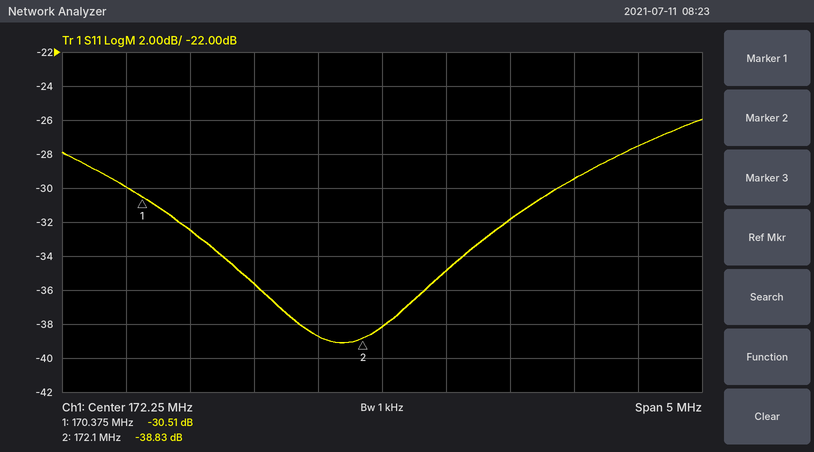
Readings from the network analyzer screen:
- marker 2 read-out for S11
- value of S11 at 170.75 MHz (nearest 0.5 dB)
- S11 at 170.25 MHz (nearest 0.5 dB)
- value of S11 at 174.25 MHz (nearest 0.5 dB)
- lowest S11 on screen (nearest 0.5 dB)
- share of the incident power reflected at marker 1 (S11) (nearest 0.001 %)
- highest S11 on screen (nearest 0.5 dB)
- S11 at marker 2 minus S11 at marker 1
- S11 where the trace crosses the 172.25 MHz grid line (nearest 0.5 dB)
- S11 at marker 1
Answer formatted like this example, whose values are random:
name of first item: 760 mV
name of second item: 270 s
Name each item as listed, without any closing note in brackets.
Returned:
marker 2 read-out for S11: -38.83 dB
value of S11 at 170.75 MHz: -32.5 dB
S11 at 170.25 MHz: -30.0 dB
value of S11 at 174.25 MHz: -27.5 dB
lowest S11 on screen: -39.0 dB
share of the incident power reflected at marker 1 (S11): 0.089 %
highest S11 on screen: -26.0 dB
S11 at marker 2 minus S11 at marker 1: -8.32 dB
S11 where the trace crosses the 172.25 MHz grid line: -38.0 dB
S11 at marker 1: -30.51 dB
